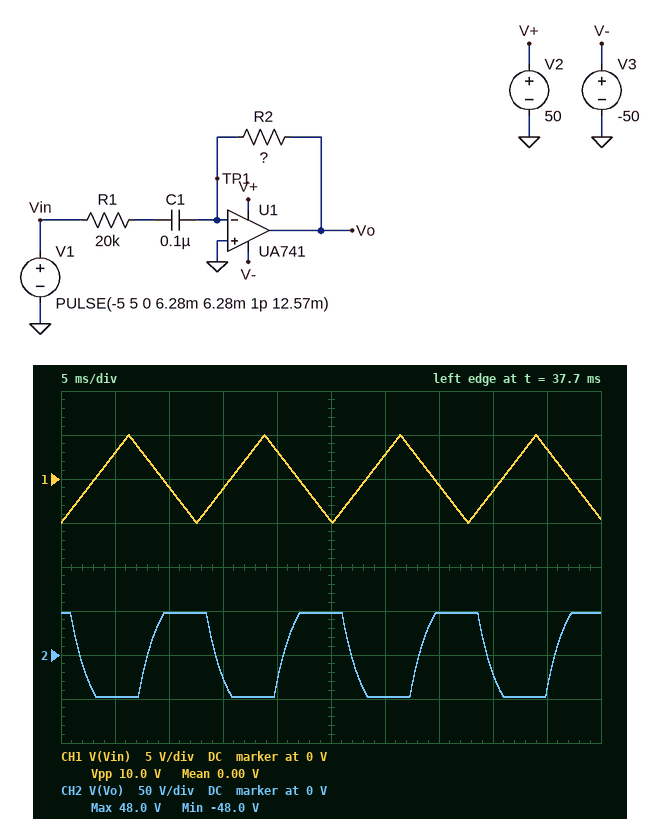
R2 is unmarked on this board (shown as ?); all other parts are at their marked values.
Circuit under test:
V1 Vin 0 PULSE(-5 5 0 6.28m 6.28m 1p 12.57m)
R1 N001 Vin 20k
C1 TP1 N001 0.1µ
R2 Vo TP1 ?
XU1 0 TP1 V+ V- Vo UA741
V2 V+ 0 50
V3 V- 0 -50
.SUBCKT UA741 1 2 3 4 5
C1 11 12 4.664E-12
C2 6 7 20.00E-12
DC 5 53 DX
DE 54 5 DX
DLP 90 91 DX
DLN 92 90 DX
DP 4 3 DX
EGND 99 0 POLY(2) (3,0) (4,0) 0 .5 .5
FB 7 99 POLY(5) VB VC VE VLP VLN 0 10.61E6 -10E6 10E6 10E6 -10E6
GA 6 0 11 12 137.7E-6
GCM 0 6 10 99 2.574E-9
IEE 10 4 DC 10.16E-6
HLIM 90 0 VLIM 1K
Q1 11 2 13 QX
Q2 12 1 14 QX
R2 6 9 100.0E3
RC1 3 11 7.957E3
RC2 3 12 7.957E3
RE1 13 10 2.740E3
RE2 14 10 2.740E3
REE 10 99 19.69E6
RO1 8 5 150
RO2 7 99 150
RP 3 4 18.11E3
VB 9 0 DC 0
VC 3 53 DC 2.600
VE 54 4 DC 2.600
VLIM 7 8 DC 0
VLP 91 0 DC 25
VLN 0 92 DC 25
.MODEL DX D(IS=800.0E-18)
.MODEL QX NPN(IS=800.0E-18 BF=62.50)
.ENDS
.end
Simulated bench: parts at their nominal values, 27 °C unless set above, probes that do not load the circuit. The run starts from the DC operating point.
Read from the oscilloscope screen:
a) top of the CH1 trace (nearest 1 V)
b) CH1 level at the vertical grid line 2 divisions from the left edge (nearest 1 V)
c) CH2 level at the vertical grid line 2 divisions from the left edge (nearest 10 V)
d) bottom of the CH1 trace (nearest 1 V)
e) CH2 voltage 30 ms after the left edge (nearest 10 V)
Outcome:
5 V
-1 V
50 V
-5 V
-50 V
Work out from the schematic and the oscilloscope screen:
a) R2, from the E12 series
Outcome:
560 kΩ
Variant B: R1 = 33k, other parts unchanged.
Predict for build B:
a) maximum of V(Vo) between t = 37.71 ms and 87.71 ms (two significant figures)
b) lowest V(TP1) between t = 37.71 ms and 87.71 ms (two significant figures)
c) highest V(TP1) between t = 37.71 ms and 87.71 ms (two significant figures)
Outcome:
48 V
-1.2 V
1.2 V
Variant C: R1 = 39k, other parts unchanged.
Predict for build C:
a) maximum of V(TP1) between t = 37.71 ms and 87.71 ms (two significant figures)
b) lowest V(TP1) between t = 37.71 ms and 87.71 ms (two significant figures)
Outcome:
830 mV
-830 mV
